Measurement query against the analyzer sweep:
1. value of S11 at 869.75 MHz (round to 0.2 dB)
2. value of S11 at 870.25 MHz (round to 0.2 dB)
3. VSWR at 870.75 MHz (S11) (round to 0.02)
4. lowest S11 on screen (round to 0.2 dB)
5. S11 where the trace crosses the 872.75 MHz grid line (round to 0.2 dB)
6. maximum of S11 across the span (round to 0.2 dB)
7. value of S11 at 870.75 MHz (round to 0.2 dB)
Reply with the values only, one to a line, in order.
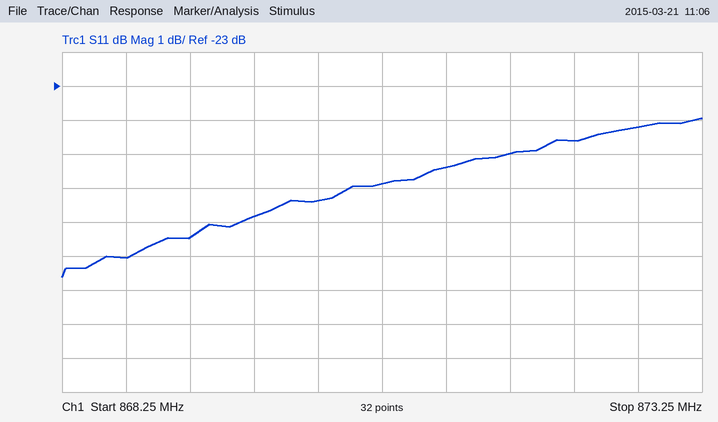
-26.8 dB
-26.4 dB
1.10
-28.6 dB
-24.2 dB
-24.0 dB
-25.8 dB
